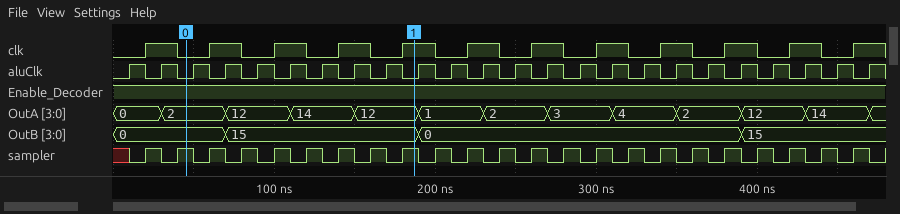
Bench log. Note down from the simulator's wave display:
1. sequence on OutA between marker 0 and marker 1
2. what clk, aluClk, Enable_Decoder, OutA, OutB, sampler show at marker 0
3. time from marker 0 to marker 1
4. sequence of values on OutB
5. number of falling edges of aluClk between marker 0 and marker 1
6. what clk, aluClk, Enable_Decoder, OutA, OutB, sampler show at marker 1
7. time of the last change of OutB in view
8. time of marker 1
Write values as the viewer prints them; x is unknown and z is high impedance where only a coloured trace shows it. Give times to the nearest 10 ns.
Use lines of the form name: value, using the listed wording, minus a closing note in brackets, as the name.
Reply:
sequence on OutA between marker 0 and marker 1: 2, 12, 14, 12
what clk, aluClk, Enable_Decoder, OutA, OutB, sampler show at marker 0: clk=0, aluClk=0, Enable_Decoder=1, OutA=2, OutB=0, sampler=1
time from marker 0 to marker 1: 140 ns
sequence of values on OutB: 0, 15, 0, 15
number of falling edges of aluClk between marker 0 and marker 1: 7
what clk, aluClk, Enable_Decoder, OutA, OutB, sampler show at marker 1: clk=1, aluClk=0, Enable_Decoder=1, OutA=12, OutB=15, sampler=1
time of the last change of OutB in view: 390 ns
time of marker 1: 190 ns
